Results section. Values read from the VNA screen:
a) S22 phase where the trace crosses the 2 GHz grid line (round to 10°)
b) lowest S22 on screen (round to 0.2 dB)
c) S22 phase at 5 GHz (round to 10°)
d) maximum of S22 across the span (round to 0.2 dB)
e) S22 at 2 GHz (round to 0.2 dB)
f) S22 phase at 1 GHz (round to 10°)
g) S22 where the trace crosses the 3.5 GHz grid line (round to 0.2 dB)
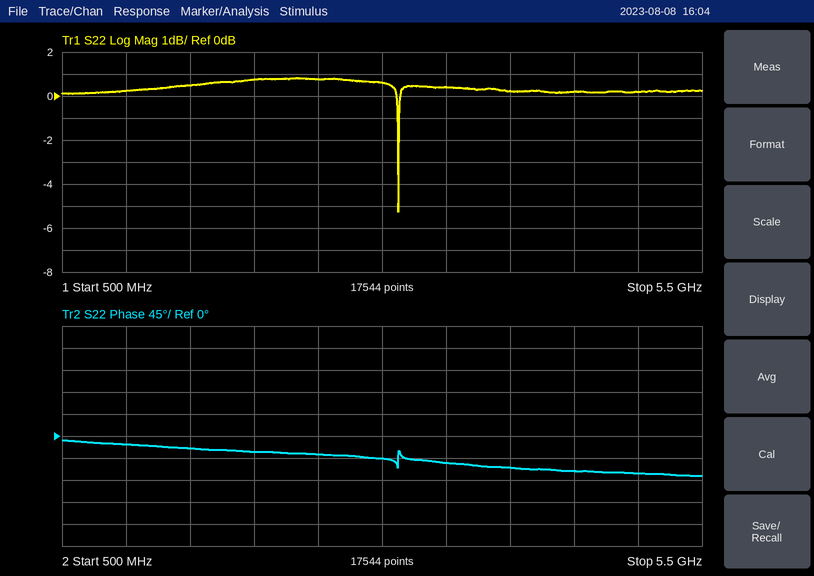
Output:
-30°
-5.2 dB
-80°
0.8 dB
0.8 dB
-20°
0.4 dB
